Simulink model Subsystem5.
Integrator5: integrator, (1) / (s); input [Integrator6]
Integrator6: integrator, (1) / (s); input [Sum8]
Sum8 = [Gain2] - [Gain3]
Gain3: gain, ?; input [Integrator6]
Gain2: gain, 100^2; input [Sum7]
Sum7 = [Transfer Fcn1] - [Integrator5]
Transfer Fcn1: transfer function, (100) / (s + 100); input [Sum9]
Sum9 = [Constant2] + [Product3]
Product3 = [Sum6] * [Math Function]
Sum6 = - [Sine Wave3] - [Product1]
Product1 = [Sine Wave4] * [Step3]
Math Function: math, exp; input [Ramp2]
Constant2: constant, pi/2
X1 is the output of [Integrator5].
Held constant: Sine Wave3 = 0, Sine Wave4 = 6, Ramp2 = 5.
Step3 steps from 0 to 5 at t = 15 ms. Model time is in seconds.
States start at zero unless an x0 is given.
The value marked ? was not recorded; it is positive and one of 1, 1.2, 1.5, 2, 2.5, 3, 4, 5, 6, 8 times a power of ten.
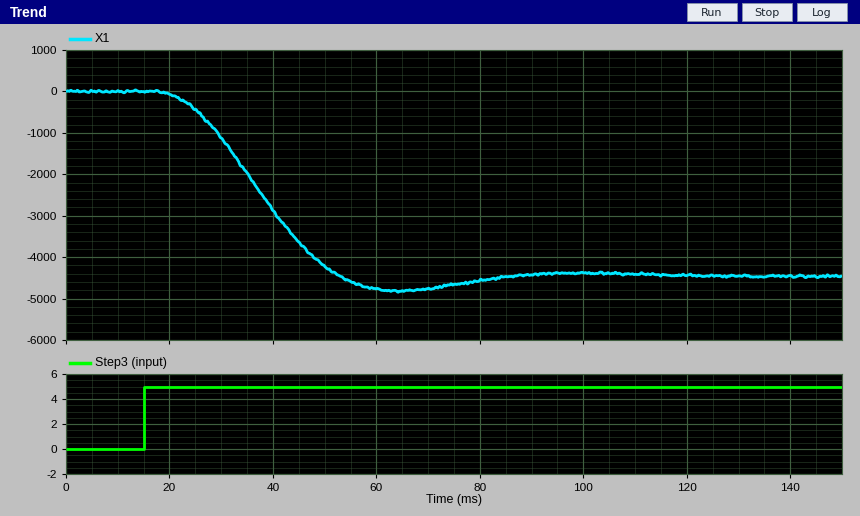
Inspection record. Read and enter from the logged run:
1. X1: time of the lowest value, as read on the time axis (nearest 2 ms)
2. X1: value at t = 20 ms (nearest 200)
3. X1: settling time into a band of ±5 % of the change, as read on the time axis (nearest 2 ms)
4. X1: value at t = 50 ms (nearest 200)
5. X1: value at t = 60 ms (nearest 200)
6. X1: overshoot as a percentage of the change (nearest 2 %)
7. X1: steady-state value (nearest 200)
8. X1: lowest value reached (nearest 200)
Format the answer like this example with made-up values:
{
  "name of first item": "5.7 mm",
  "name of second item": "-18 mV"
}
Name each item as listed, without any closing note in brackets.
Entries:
{
  "X1: time of the lowest value, as read on the time axis": "64 ms",
  "X1: value at t = 20 ms": "0",
  "X1: settling time into a band of ±5 % of the change, as read on the time axis": "74 ms",
  "X1: value at t = 50 ms": "-4200",
  "X1: value at t = 60 ms": "-4800",
  "X1: overshoot as a percentage of the change": "8 %",
  "X1: steady-state value": "-4400",
  "X1: lowest value reached": "-4800"
}
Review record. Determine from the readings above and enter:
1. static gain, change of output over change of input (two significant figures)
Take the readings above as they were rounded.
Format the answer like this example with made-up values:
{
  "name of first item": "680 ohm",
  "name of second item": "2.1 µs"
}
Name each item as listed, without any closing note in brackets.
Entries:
{
  "static gain, change of output over change of input": "-880"
}
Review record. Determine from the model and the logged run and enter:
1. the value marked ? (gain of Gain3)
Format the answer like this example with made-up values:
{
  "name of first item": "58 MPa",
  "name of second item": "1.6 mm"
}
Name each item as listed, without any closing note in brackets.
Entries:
{
  "the value marked ?": "100"
}
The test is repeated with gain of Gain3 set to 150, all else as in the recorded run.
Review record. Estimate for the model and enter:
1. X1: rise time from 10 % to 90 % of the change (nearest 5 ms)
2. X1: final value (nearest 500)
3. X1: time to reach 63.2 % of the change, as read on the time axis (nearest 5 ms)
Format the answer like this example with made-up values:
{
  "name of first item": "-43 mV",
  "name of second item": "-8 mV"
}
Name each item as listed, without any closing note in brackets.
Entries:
{
  "X1: rise time from 10 % to 90 % of the change": "30 ms",
  "X1: final value": "-4500",
  "X1: time to reach 63.2 % of the change, as read on the time axis": "45 ms"
}
